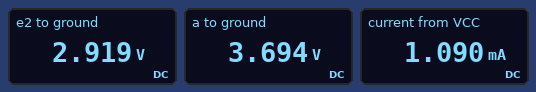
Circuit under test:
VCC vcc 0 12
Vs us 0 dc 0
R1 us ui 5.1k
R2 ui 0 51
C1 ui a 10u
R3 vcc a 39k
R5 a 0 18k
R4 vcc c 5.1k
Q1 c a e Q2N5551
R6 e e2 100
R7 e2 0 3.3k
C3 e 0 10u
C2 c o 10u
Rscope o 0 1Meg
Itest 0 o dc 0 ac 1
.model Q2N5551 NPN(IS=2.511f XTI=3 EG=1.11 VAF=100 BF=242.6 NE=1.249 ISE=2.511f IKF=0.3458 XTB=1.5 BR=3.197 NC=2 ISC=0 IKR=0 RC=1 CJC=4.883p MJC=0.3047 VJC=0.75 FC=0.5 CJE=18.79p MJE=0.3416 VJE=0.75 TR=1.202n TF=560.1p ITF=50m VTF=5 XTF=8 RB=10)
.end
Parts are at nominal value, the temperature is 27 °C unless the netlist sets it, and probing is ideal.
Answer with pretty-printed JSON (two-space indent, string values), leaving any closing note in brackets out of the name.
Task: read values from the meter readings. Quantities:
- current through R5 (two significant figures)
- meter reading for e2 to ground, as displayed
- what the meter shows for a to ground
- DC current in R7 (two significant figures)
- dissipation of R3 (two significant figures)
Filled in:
{
  "current through R5": "210 µA",
  "meter reading for e2 to ground, as displayed": "2.919 V",
  "what the meter shows for a to ground": "3.694 V",
  "DC current in R7": "880 µA",
  "dissipation of R3": "1.8 mW"
}
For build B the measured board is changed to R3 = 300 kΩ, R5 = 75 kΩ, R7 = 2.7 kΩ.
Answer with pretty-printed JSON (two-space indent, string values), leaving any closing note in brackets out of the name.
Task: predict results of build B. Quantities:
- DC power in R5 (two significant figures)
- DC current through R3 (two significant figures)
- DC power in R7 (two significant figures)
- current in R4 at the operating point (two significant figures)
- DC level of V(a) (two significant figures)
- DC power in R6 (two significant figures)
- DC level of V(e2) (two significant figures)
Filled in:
{
  "DC power in R5": "60 µW",
  "DC current through R3": "33 µA",
  "DC power in R7": "720 µW",
  "current in R4 at the operating point": "510 µA",
  "DC level of V(a)": "2.1 V",
  "DC power in R6": "27 µW",
  "DC level of V(e2)": "1.4 V"
}
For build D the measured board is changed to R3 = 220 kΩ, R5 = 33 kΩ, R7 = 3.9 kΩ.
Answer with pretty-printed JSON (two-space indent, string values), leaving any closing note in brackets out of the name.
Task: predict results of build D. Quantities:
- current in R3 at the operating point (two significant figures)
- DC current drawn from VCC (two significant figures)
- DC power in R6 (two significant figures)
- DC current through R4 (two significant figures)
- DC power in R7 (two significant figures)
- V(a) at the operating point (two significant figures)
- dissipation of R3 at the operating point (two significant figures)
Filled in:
{
  "current in R3 at the operating point": "48 µA",
  "DC current drawn from VCC": "260 µA",
  "DC power in R6": "4.6 µW",
  "DC current through R4": "210 µA",
  "DC power in R7": "180 µW",
  "V(a) at the operating point": "1.5 V",
  "dissipation of R3 at the operating point": "500 µW"
}
